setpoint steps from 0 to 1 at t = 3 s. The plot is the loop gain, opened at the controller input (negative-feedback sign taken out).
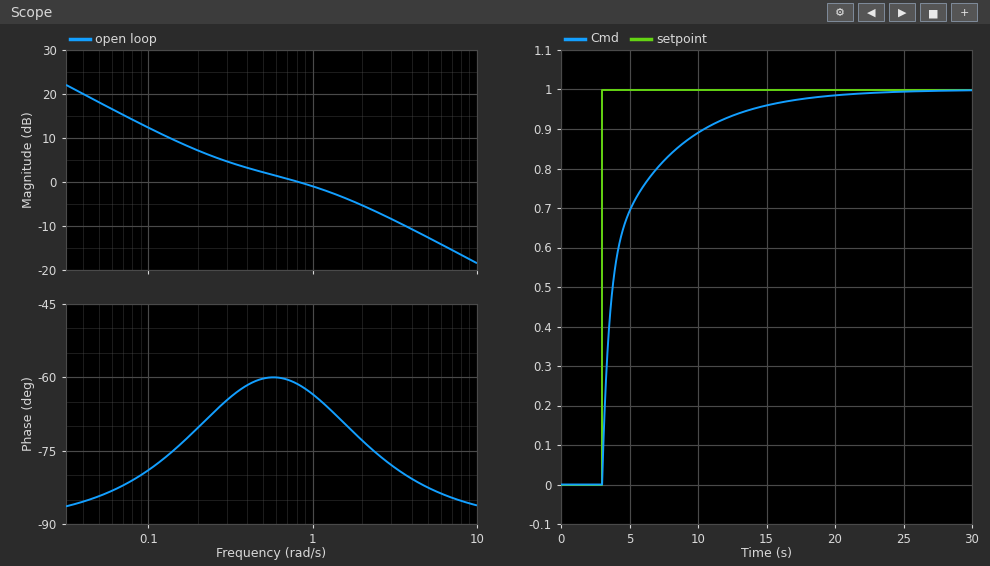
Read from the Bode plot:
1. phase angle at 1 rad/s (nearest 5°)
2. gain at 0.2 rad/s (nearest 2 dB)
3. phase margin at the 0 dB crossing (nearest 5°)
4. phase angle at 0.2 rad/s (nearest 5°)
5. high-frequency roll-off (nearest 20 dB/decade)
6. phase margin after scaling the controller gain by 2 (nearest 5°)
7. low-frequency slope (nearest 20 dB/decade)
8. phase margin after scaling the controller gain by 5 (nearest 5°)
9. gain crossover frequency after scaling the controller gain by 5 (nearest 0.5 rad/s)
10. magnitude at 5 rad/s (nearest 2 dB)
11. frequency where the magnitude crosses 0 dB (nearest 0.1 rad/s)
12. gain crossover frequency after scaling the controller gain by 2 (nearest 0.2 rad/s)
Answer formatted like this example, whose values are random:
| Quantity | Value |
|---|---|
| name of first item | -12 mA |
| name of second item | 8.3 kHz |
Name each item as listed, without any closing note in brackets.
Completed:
| Quantity | Value |
|---|---|
| phase angle at 1 rad/s | -65° |
| gain at 0.2 rad/s | 8 dB |
| phase margin at the 0 dB crossing | 120° |
| phase angle at 0.2 rad/s | -70° |
| high-frequency roll-off | -20 dB/decade |
| phase margin after scaling the controller gain by 2 | 105° |
| low-frequency slope | -20 dB/decade |
| phase margin after scaling the controller gain by 5 | 95° |
| gain crossover frequency after scaling the controller gain by 5 | 6.0 rad/s |
| magnitude at 5 rad/s | -12 dB |
| frequency where the magnitude crosses 0 dB | 0.8 rad/s |
| gain crossover frequency after scaling the controller gain by 2 | 2.2 rad/s |
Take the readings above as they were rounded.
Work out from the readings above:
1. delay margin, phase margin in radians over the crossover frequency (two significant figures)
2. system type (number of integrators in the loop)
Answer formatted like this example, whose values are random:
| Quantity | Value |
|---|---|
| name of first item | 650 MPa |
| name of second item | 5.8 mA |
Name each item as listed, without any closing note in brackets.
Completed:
| Quantity | Value |
|---|---|
| delay margin, phase margin in radians over the crossover frequency | 2.6 s |
| system type | 1 |
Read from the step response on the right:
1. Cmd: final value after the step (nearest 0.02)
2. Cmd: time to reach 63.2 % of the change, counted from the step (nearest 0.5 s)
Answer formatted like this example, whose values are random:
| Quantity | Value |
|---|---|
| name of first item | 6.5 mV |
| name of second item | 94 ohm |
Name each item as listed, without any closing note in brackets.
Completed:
| Quantity | Value |
|---|---|
| Cmd: final value after the step | 1.00 |
| Cmd: time to reach 63.2 % of the change, counted from the step | 1.5 s |
